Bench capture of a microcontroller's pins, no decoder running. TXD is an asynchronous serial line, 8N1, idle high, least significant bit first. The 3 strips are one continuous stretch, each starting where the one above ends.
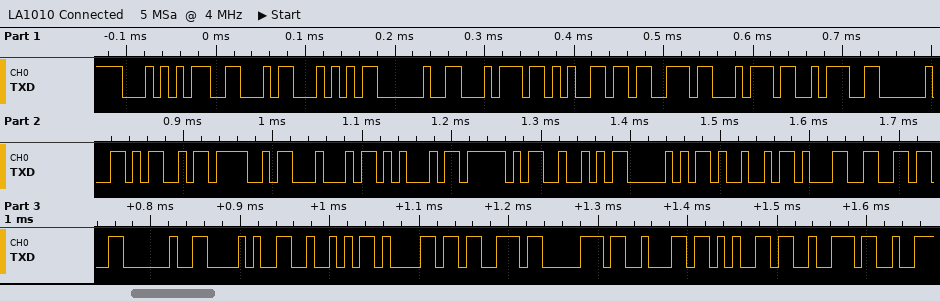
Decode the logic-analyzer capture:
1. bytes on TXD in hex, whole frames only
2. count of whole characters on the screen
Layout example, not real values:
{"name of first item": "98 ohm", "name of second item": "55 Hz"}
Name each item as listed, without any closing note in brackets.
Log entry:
{"bytes on TXD in hex, whole frames only": "54 46 54 20 74 65 73 74 3A 20 4D 4F 44 45 5F 52 50 49 31 36 20 28 52 61 73 70 62 65 72", "count of whole characters on the screen": "29"}
